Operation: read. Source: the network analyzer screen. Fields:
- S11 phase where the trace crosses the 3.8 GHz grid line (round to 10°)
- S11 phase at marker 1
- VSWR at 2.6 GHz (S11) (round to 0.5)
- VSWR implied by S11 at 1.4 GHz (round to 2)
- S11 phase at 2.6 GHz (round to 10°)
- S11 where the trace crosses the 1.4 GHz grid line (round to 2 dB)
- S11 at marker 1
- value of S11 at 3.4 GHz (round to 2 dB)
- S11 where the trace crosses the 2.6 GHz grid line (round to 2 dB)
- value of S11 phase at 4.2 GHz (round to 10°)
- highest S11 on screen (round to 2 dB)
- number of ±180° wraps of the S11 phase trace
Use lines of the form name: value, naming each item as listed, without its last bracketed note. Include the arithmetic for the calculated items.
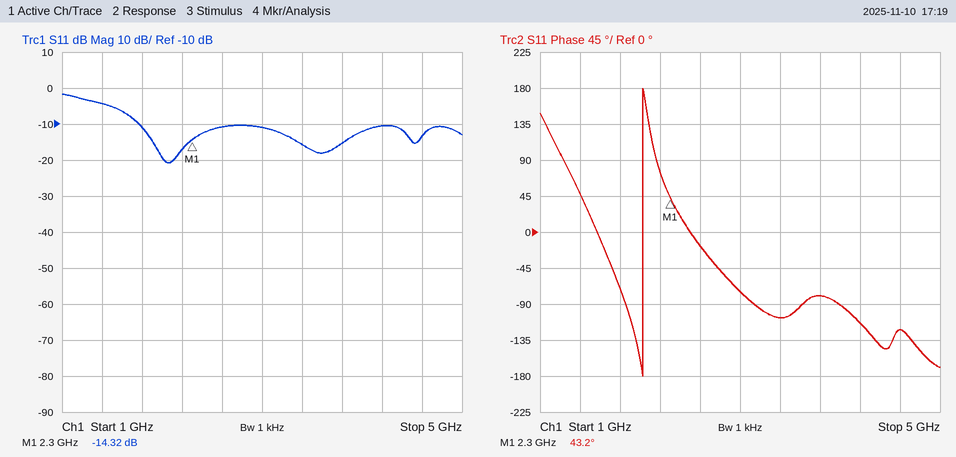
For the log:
S11 phase where the trace crosses the 3.8 GHz grid line: -80°
S11 phase at marker 1: 43.2°
VSWR at 2.6 GHz (S11): |Γ| = 10^(-10/20) = 0.3162; VSWR = (1 + 0.3162)/(1 − 0.3162) ≈ 1.92, so 2.0 to the nearest 0.5
VSWR implied by S11 at 1.4 GHz: |Γ| = 10^(-4/20) = 0.6310; VSWR = (1 + 0.6310)/(1 − 0.6310) ≈ 4
S11 phase at 2.6 GHz: -20°
S11 where the trace crosses the 1.4 GHz grid line: -4 dB
S11 at marker 1: -14.32 dB
value of S11 at 3.4 GHz: -16 dB
S11 where the trace crosses the 2.6 GHz grid line: -10 dB
value of S11 phase at 4.2 GHz: -110°
highest S11 on screen: -2 dB
number of ±180° wraps of the S11 phase trace: 1
